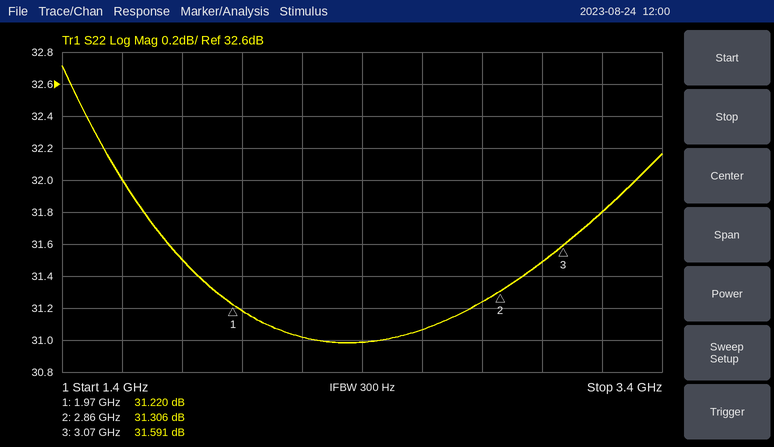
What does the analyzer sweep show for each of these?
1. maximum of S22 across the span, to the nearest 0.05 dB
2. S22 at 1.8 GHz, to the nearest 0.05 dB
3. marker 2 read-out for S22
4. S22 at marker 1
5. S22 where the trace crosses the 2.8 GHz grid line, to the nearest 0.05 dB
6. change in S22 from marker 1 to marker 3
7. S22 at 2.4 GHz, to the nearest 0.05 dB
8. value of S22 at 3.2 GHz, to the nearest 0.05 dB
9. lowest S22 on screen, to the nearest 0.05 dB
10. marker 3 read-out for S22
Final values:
32.70 dB
31.50 dB
31.306 dB
31.220 dB
31.25 dB
0.371 dB
31.00 dB
31.80 dB
31.00 dB
31.591 dB
